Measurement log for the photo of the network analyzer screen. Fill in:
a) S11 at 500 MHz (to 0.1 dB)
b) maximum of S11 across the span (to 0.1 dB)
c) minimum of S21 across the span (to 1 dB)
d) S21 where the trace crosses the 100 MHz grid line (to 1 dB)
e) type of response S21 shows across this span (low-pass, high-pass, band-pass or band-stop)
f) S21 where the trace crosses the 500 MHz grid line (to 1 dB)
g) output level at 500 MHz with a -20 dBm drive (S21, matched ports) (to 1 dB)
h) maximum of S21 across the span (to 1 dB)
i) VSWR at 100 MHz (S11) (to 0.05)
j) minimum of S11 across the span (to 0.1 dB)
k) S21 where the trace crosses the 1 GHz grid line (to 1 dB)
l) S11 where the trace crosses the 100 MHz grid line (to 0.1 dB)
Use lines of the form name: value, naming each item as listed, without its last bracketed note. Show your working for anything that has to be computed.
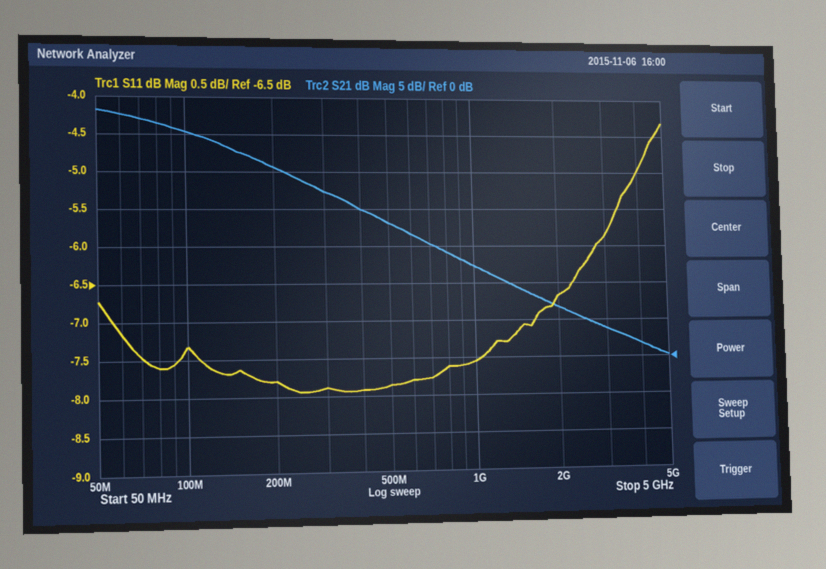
S11 at 500 MHz: -7.9 dB
maximum of S11 across the span: -4.3 dB
minimum of S21 across the span: 0 dB
S21 where the trace crosses the 100 MHz grid line: 30 dB
type of response S21 shows across this span: low-pass
S21 where the trace crosses the 500 MHz grid line: 18 dB
output level at 500 MHz with a -20 dBm drive (S21, matched ports): -20 dBm + (18 dB) = -2 dBm
maximum of S21 across the span: 33 dB
VSWR at 100 MHz (S11): |Γ| = 10^(-7.3/20) = 0.4315; VSWR = (1 + 0.4315)/(1 − 0.4315) ≈ 2.52, so 2.50 to the nearest 0.05
minimum of S11 across the span: -7.9 dB
S21 where the trace crosses the 1 GHz grid line: 12 dB
S11 where the trace crosses the 100 MHz grid line: -7.3 dB
